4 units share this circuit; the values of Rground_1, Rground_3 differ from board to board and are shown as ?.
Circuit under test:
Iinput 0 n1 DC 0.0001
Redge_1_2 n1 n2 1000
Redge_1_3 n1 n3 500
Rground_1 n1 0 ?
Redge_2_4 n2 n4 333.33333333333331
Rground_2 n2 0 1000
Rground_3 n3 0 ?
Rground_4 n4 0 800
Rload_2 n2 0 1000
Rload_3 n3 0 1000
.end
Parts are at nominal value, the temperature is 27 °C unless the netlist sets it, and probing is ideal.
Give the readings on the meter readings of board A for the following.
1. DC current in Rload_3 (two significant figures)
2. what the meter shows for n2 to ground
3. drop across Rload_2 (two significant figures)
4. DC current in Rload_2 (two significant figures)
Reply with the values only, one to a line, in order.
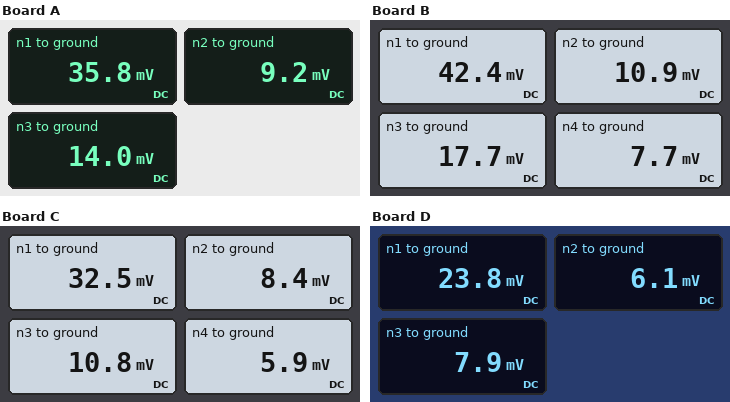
14 µA
9.2 mV
9.2 mV
9.2 µA
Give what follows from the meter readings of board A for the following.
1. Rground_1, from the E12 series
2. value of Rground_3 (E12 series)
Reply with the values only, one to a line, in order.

1.2 kΩ
470 Ω
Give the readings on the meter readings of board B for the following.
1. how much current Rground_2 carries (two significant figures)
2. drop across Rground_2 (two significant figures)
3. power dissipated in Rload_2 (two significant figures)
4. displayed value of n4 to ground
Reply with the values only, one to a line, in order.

11 µA
11 mV
120 nW
7.7 mV
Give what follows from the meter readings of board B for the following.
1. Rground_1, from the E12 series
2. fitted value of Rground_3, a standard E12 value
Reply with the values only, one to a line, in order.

2.2 kΩ
560 Ω
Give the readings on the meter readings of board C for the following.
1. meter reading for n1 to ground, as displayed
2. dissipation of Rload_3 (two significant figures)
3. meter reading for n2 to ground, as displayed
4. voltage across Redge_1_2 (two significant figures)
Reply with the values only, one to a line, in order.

32.5 mV
120 nW
8.4 mV
24 mV
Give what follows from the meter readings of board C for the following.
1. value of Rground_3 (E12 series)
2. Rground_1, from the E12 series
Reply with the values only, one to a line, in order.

330 Ω
1 kΩ
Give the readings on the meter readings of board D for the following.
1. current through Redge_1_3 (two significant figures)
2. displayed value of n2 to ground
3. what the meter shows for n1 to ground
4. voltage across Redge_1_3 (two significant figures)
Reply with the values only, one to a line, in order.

32 µA
6.1 mV
23.8 mV
16 mV
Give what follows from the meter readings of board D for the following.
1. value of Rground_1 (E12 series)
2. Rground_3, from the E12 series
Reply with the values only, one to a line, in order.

470 Ω
330 Ω
